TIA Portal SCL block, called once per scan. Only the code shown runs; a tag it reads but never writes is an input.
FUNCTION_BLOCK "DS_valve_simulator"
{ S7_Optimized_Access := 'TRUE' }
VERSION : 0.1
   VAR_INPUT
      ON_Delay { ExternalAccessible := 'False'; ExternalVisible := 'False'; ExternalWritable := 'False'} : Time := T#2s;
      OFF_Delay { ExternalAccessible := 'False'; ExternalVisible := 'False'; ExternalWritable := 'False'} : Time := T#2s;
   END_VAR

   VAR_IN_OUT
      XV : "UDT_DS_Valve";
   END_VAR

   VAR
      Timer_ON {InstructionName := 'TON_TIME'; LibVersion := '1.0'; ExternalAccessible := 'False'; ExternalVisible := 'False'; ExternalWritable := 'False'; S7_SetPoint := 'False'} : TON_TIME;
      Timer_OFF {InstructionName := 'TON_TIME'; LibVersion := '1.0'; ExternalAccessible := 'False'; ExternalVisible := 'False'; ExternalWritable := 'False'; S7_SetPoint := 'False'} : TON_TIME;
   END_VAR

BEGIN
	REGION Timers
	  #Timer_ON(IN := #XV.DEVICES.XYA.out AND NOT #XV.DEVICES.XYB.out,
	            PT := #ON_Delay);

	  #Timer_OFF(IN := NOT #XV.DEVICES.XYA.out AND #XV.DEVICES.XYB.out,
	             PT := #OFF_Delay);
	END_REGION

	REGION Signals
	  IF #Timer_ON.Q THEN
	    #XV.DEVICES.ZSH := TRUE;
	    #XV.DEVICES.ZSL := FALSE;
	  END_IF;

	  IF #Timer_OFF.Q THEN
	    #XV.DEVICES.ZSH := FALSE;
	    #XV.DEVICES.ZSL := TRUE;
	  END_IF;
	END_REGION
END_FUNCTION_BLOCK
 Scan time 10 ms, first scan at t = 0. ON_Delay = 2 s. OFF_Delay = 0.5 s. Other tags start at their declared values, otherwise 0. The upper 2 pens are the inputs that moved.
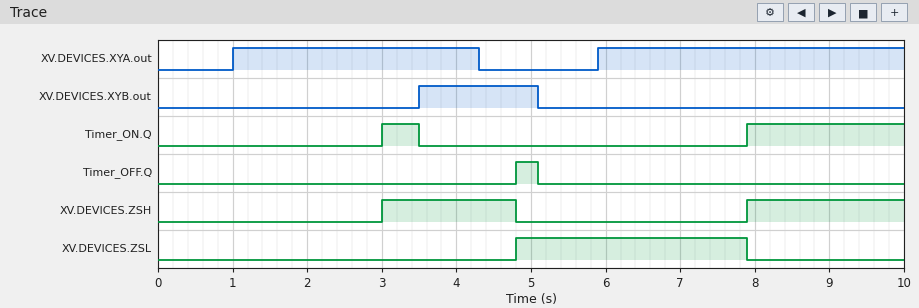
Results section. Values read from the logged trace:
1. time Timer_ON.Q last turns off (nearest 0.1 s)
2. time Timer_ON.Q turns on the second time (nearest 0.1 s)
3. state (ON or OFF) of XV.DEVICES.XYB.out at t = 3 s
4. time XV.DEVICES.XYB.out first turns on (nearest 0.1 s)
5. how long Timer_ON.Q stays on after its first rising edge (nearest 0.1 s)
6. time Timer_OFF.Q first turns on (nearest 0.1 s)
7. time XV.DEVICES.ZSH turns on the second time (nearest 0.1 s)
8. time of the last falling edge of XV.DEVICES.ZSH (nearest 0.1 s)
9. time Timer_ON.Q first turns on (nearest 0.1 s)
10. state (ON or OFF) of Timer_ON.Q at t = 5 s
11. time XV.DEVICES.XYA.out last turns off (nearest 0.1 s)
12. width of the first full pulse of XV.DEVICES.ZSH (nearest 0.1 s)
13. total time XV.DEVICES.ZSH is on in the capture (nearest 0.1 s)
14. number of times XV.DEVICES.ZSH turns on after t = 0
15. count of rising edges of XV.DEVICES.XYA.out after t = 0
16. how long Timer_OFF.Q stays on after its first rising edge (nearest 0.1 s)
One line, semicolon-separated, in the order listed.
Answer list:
3.5 s; 7.9 s; OFF; 3.5 s; 0.5 s; 4.8 s; 7.9 s; 4.8 s; 3.0 s; OFF; 4.3 s; 1.8 s; 3.9 s; 2; 2; 0.3 s
